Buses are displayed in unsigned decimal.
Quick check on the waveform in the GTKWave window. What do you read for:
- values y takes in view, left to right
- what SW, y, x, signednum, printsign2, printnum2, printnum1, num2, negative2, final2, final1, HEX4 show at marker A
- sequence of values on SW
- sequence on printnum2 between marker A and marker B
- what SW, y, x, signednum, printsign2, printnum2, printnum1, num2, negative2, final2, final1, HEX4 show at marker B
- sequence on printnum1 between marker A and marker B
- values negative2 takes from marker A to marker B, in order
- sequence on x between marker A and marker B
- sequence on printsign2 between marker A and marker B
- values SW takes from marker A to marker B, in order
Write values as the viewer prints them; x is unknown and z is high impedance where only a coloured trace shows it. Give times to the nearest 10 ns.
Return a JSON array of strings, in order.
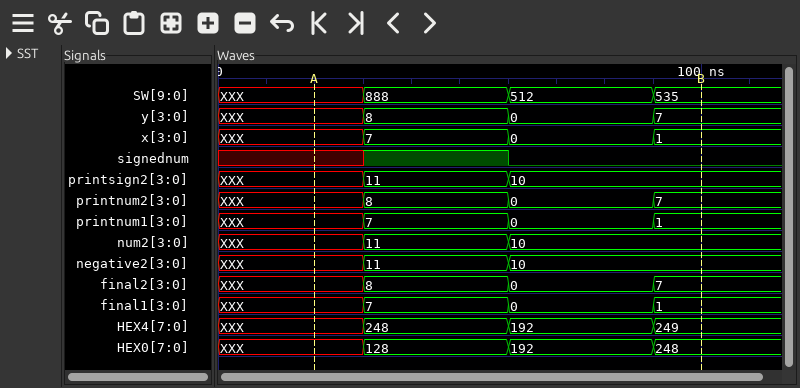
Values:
["XXX, 8, 0, 7", "SW=XXX, y=XXX, x=XXX, signednum=x, printsign2=XXX, printnum2=XXX, printnum1=XXX, num2=XXX, negative2=XXX, final2=XXX, final1=XXX, HEX4=XXX", "XXX, 888, 512, 535", "XXX, 8, 0, 7", "SW=535, y=7, x=1, signednum=0, printsign2=10, printnum2=7, printnum1=1, num2=10, negative2=10, final2=7, final1=1, HEX4=249", "XXX, 7, 0, 1", "XXX, 11, 10", "XXX, 7, 0, 1", "XXX, 11, 10", "XXX, 888, 512, 535"]
